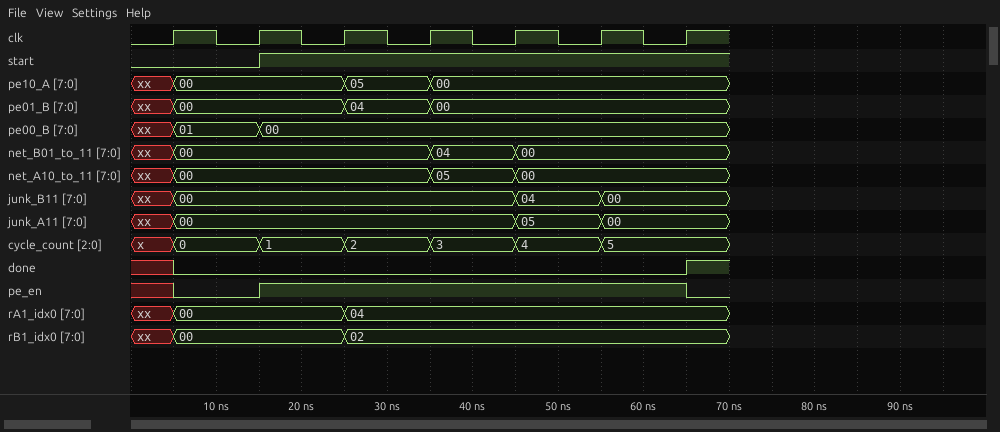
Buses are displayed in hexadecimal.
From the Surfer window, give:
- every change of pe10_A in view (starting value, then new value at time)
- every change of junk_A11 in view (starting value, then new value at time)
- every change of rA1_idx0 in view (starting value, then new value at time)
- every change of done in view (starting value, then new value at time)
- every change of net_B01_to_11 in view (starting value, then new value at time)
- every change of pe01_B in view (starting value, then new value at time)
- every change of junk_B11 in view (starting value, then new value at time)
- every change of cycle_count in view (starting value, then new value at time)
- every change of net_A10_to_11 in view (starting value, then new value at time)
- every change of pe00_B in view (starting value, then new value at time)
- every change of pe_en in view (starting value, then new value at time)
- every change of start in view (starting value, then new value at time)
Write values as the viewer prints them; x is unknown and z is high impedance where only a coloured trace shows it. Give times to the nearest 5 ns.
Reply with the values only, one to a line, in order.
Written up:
xx, 00 at 5 ns, 05 at 25 ns, 00 at 35 ns
xx, 00 at 5 ns, 05 at 45 ns, 00 at 55 ns
xx, 00 at 5 ns, 04 at 25 ns
x, 0 at 5 ns, 1 at 65 ns
xx, 00 at 5 ns, 04 at 35 ns, 00 at 45 ns
xx, 00 at 5 ns, 04 at 25 ns, 00 at 35 ns
xx, 00 at 5 ns, 04 at 45 ns, 00 at 55 ns
x, 0 at 5 ns, 1 at 15 ns, 2 at 25 ns, 3 at 35 ns, 4 at 45 ns, 5 at 55 ns
xx, 00 at 5 ns, 05 at 35 ns, 00 at 45 ns
xx, 01 at 5 ns, 00 at 15 ns
x, 0 at 5 ns, 1 at 15 ns, 0 at 65 ns
0, 1 at 15 ns
